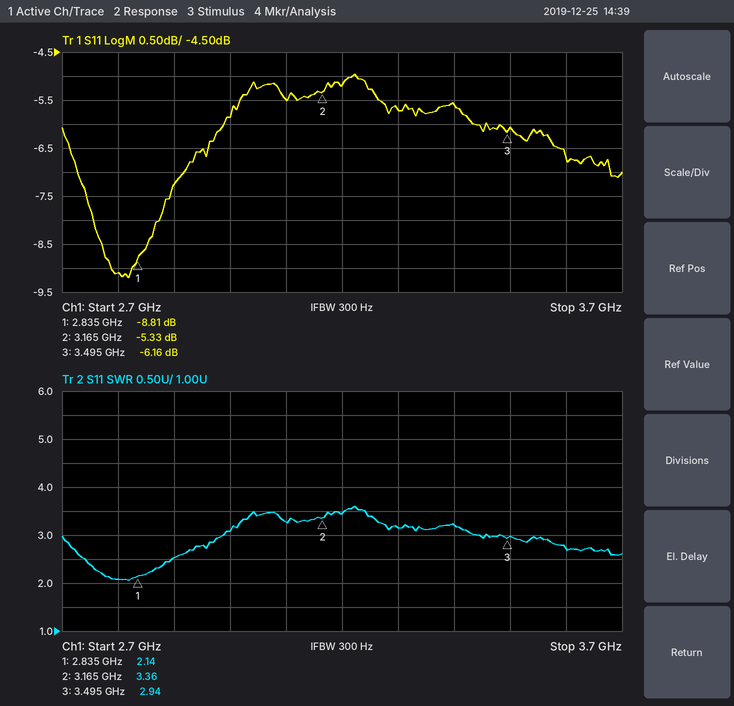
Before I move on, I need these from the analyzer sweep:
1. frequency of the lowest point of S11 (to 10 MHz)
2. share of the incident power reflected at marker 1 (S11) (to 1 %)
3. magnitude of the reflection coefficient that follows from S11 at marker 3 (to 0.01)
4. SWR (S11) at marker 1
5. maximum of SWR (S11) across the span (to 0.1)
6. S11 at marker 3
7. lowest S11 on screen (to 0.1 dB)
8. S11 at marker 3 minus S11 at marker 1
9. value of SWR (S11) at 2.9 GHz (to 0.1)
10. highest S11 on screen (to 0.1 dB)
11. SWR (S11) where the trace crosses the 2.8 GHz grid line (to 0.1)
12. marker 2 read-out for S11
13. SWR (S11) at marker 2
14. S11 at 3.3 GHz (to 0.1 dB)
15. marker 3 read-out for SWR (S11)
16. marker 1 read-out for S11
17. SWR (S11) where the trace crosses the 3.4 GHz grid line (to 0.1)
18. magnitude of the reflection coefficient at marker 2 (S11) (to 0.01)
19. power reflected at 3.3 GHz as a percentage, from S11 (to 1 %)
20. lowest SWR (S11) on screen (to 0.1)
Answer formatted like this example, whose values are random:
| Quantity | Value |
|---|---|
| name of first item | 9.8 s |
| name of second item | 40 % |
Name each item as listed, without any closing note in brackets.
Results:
| Quantity | Value |
|---|---|
| frequency of the lowest point of S11 | 2.82 GHz |
| share of the incident power reflected at marker 1 (S11) | 13 % |
| magnitude of the reflection coefficient that follows from S11 at marker 3 | 0.49 |
| SWR (S11) at marker 1 | 2.14 |
| maximum of SWR (S11) across the span | 3.6 |
| S11 at marker 3 | -6.16 dB |
| lowest S11 on screen | -9.2 dB |
| S11 at marker 3 minus S11 at marker 1 | 2.65 dB |
| value of SWR (S11) at 2.9 GHz | 2.5 |
| highest S11 on screen | -5.0 dB |
| SWR (S11) where the trace crosses the 2.8 GHz grid line | 2.1 |
| marker 2 read-out for S11 | -5.33 dB |
| SWR (S11) at marker 2 | 3.36 |
| S11 at 3.3 GHz | -5.7 dB |
| marker 3 read-out for SWR | 2.94 |
| marker 1 read-out for S11 | -8.81 dB |
| SWR (S11) where the trace crosses the 3.4 GHz grid line | 3.2 |
| magnitude of the reflection coefficient at marker 2 (S11) | 0.54 |
| power reflected at 3.3 GHz as a percentage, from S11 | 27 % |
| lowest SWR (S11) on screen | 2.1 |
